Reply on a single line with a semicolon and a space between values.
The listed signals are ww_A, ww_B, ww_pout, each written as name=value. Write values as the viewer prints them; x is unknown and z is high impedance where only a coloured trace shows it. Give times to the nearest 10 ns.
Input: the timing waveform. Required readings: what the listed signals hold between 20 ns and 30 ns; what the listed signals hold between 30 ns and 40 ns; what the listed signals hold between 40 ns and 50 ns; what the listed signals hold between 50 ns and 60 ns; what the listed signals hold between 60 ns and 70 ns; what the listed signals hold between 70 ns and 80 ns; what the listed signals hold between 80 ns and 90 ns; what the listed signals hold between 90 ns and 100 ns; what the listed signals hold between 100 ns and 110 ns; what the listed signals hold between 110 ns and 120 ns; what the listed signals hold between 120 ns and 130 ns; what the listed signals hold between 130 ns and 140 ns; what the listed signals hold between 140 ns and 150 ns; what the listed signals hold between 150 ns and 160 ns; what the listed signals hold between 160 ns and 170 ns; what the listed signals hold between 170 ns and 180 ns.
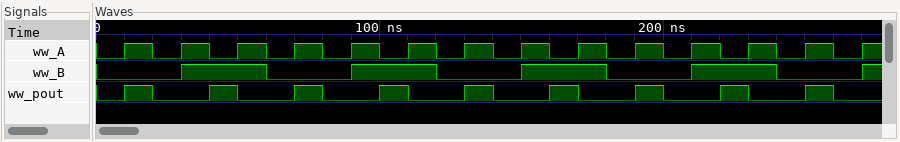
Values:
ww_A=0, ww_B=0, ww_pout=0; ww_A=1, ww_B=1, ww_pout=0; ww_A=0, ww_B=1, ww_pout=1; ww_A=1, ww_B=1, ww_pout=0; ww_A=0, ww_B=0, ww_pout=0; ww_A=1, ww_B=0, ww_pout=1; ww_A=0, ww_B=0, ww_pout=0; ww_A=1, ww_B=1, ww_pout=0; ww_A=0, ww_B=1, ww_pout=1; ww_A=1, ww_B=1, ww_pout=0; ww_A=0, ww_B=0, ww_pout=0; ww_A=1, ww_B=0, ww_pout=1; ww_A=0, ww_B=0, ww_pout=0; ww_A=1, ww_B=1, ww_pout=0; ww_A=0, ww_B=1, ww_pout=1; ww_A=1, ww_B=1, ww_pout=0
